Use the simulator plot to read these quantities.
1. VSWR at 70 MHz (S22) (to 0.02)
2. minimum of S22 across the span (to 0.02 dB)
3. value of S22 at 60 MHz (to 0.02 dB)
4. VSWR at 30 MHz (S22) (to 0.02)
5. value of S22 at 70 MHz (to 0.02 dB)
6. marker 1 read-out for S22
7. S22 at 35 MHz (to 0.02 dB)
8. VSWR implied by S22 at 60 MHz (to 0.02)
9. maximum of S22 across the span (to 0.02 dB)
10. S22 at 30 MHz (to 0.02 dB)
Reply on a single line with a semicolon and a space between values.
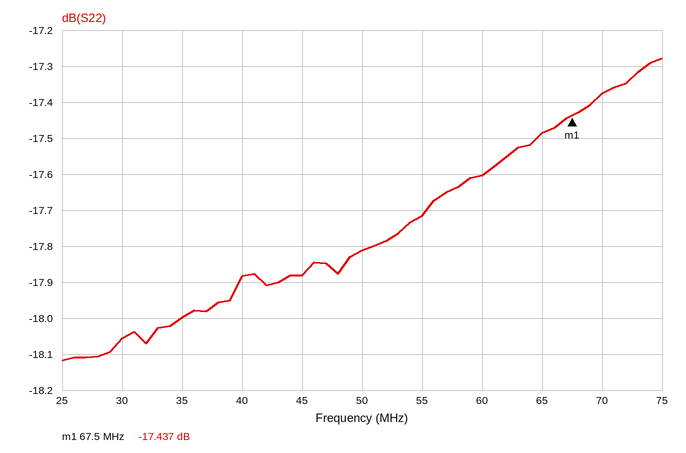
1.32; -18.12 dB; -17.60 dB; 1.28; -17.38 dB; -17.437 dB; -18.00 dB; 1.30; -17.28 dB; -18.06 dB
